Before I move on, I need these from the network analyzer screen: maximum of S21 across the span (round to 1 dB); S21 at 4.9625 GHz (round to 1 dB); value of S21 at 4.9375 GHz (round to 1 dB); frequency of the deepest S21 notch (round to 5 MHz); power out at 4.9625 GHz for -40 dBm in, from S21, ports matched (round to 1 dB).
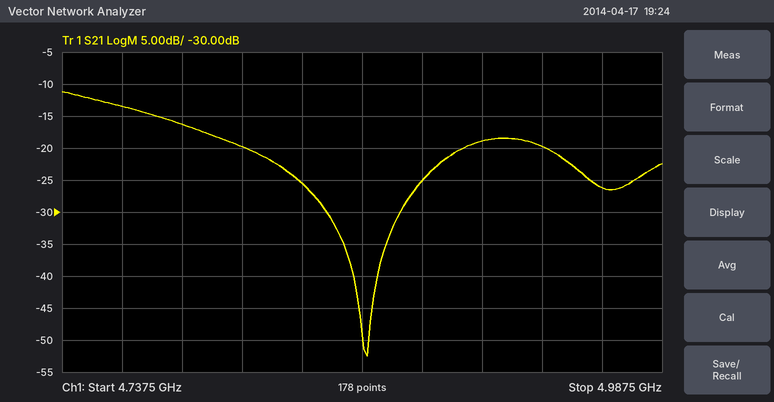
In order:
-11 dB
-26 dB
-20 dB
4.865 GHz
-66 dBm
